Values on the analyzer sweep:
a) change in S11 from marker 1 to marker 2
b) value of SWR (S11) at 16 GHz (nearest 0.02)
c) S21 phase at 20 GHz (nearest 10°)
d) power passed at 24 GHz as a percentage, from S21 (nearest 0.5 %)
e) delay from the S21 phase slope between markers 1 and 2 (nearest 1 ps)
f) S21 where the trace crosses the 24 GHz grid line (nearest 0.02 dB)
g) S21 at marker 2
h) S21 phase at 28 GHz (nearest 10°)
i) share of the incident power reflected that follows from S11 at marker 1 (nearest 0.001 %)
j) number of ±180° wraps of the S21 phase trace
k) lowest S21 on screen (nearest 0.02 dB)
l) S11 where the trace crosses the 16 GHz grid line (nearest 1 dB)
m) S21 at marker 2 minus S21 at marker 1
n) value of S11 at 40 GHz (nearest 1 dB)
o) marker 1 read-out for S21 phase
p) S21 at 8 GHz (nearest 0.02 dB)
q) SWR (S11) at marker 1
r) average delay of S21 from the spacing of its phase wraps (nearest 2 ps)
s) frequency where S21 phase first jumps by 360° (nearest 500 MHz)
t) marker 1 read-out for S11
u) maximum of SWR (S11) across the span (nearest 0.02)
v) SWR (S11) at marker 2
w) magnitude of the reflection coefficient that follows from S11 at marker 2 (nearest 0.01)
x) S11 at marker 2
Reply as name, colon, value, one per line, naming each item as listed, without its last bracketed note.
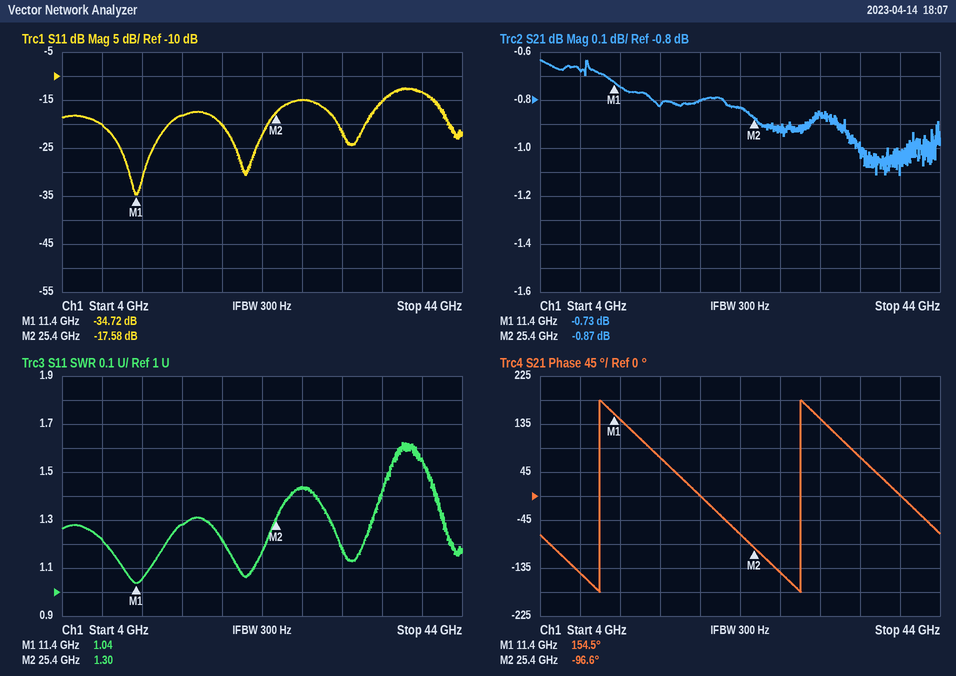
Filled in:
change in S11 from marker 1 to marker 2: 17.14 dB
value of SWR (S11) at 16 GHz: 1.28
S21 phase at 20 GHz: 0°
power passed at 24 GHz as a percentage, from S21: 82.5 %
delay from the S21 phase slope between markers 1 and 2: 50 ps
S21 where the trace crosses the 24 GHz grid line: -0.84 dB
S21 at marker 2: -0.87 dB
S21 phase at 28 GHz: -140°
share of the incident power reflected that follows from S11 at marker 1: 0.034 %
number of ±180° wraps of the S21 phase trace: 2
lowest S21 on screen: -1.12 dB
S11 where the trace crosses the 16 GHz grid line: -18 dB
S21 at marker 2 minus S21 at marker 1: -0.14 dB
value of S11 at 40 GHz: -13 dB
marker 1 read-out for S21 phase: 154.5°
S21 at 8 GHz: -0.68 dB
SWR (S11) at marker 1: 1.04
average delay of S21 from the spacing of its phase wraps: 50 ps
frequency where S21 phase first jumps by 360°: 10.0 GHz
marker 1 read-out for S11: -34.72 dB
maximum of SWR (S11) across the span: 1.62
SWR (S11) at marker 2: 1.30
magnitude of the reflection coefficient that follows from S11 at marker 2: 0.13
S11 at marker 2: -17.58 dB
